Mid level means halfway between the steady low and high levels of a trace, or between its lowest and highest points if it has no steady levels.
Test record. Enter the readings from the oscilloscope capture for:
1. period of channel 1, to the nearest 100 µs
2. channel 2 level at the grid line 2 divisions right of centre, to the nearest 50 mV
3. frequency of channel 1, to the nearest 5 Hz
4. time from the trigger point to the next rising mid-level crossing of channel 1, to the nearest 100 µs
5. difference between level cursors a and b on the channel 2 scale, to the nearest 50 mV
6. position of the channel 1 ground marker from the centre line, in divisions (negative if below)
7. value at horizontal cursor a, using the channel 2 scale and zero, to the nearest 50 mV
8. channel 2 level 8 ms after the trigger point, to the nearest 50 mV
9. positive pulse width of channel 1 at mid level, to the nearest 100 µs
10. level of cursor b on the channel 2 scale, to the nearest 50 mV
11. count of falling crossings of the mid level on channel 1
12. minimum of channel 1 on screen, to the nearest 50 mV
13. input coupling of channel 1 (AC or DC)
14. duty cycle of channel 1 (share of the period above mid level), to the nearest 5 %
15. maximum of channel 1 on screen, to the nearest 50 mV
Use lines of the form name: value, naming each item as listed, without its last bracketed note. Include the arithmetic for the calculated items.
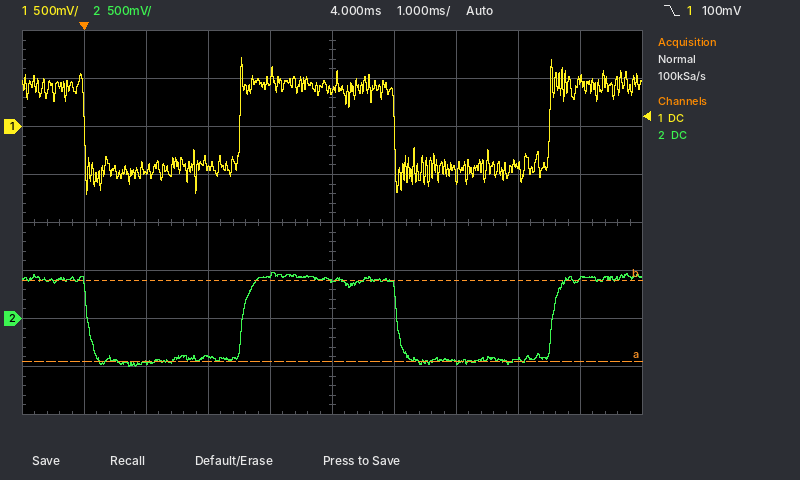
period of channel 1, to the nearest 100 µs: 5.0 ms
channel 2 level at the grid line 2 divisions right of centre, to the nearest 50 mV: -450 mV
frequency of channel 1, to the nearest 5 Hz: 1 / 5.0 ms ≈ 200 Hz
time from the trigger point to the next rising mid-level crossing of channel 1, to the nearest 100 µs: 2.5 ms
difference between level cursors a and b on the channel 2 scale, to the nearest 50 mV: 850 mV
position of the channel 1 ground marker from the centre line, in divisions: +2.0 div
value at horizontal cursor a, using the channel 2 scale and zero, to the nearest 50 mV: -450 mV
channel 2 level 8 ms after the trigger point, to the nearest 50 mV: 400 mV
positive pulse width of channel 1 at mid level, to the nearest 100 µs: 2.5 ms
level of cursor b on the channel 2 scale, to the nearest 50 mV: 400 mV
count of falling crossings of the mid level on channel 1: 2
minimum of channel 1 on screen, to the nearest 50 mV: -700 mV
input coupling of channel 1: DC
duty cycle of channel 1 (share of the period above mid level), to the nearest 5 %: 2.5 ms / 5.0 ms ≈ 50 %
maximum of channel 1 on screen, to the nearest 50 mV: 700 mV
